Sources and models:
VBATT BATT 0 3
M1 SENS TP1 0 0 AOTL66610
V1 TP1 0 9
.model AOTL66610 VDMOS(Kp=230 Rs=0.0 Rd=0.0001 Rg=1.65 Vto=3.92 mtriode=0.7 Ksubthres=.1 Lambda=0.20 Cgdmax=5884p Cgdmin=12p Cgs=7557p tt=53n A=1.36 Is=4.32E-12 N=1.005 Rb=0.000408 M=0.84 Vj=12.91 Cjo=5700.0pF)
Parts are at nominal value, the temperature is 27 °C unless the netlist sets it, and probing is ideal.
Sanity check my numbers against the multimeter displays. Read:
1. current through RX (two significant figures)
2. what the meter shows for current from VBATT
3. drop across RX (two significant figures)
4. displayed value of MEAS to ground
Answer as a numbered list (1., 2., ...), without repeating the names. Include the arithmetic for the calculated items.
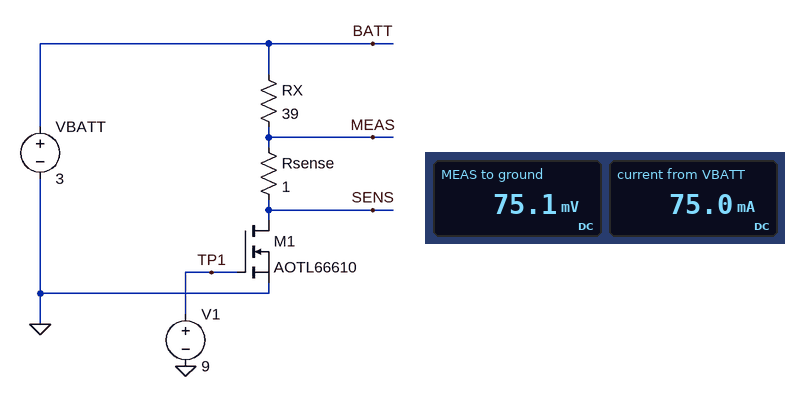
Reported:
1. (3 V - 75.1 mV) / 39 Ω = 75 mA
2. 75.0 mA
3. 3 V - 75.1 mV = 2.9 V
4. 75.1 mV
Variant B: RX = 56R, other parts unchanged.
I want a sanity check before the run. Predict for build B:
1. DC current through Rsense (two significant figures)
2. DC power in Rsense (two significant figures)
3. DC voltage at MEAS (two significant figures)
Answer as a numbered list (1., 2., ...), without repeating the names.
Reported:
1. 53 mA
2. 2.8 mW
3. 53 mV
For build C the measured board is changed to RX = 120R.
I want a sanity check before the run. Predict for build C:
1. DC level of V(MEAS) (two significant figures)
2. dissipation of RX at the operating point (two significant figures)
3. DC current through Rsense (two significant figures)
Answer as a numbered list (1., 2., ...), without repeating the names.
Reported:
1. 25 mV
2. 74 mW
3. 25 mA
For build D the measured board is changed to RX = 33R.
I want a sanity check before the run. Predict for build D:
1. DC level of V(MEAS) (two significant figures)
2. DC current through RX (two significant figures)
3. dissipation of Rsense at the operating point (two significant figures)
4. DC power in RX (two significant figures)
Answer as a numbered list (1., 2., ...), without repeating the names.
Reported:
1. 88 mV
2. 88 mA
3. 7.8 mW
4. 260 mW
